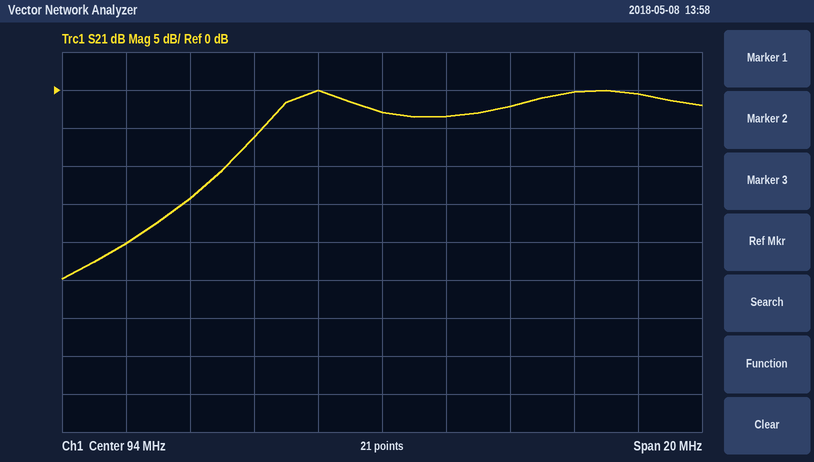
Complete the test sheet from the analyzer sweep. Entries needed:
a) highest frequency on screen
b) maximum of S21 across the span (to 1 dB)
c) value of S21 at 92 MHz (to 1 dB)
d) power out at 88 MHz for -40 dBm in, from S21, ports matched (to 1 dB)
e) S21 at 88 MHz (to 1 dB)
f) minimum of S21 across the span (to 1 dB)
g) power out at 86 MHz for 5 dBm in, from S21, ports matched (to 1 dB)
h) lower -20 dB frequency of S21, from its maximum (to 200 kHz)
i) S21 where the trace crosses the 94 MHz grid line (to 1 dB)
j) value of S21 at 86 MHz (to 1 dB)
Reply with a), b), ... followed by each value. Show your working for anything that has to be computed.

a) 104 MHz
b) 0 dB
c) 0 dB
d) -40 dBm + (-14 dB) = -54 dBm
e) -14 dB
f) -25 dB
g) 5 dBm + (-20 dB) = -15 dBm
h) 86.0 MHz
i) -3 dB
j) -20 dB
